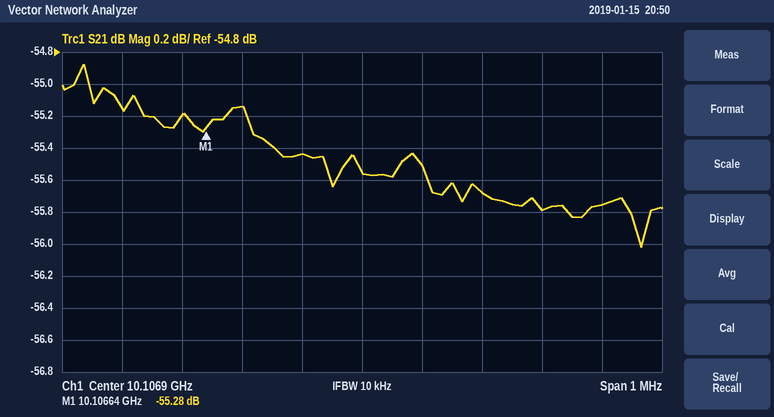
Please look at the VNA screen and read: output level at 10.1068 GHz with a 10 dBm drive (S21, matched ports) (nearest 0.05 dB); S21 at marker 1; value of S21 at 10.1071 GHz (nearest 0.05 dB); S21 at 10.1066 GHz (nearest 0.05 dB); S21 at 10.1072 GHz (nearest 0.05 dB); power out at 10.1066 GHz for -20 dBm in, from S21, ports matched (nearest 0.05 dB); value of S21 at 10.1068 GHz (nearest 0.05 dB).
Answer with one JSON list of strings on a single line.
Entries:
["-45.45 dBm", "-55.28 dB", "-55.70 dB", "-55.20 dB", "-55.80 dB", "-75.20 dBm", "-55.45 dB"]
